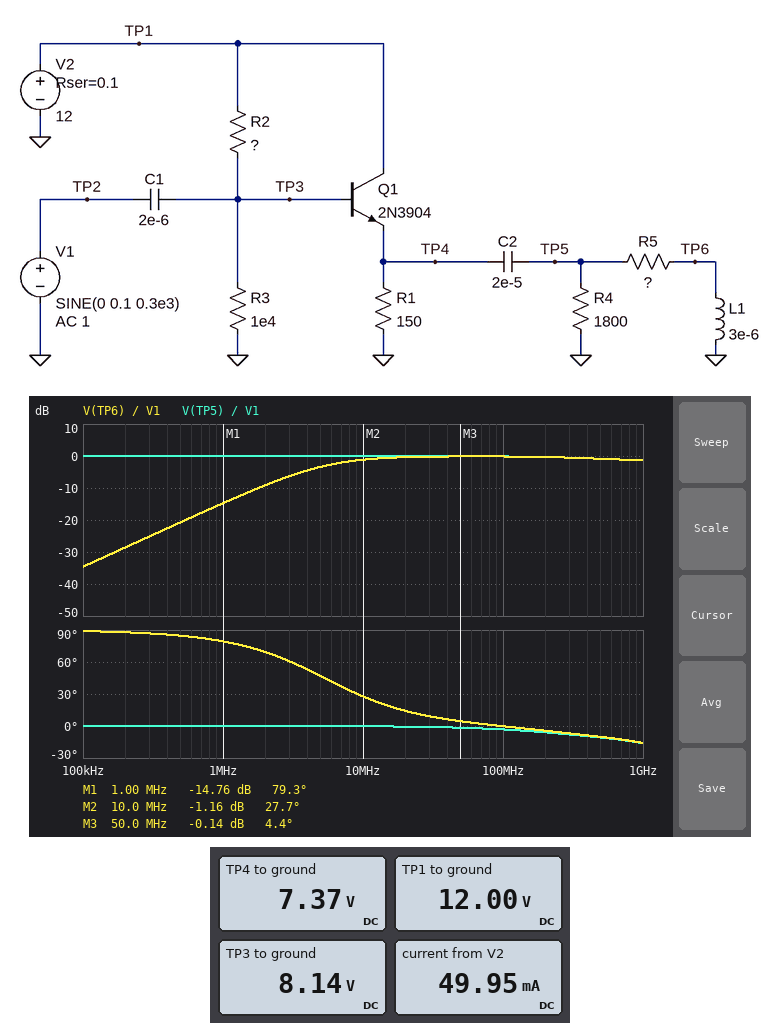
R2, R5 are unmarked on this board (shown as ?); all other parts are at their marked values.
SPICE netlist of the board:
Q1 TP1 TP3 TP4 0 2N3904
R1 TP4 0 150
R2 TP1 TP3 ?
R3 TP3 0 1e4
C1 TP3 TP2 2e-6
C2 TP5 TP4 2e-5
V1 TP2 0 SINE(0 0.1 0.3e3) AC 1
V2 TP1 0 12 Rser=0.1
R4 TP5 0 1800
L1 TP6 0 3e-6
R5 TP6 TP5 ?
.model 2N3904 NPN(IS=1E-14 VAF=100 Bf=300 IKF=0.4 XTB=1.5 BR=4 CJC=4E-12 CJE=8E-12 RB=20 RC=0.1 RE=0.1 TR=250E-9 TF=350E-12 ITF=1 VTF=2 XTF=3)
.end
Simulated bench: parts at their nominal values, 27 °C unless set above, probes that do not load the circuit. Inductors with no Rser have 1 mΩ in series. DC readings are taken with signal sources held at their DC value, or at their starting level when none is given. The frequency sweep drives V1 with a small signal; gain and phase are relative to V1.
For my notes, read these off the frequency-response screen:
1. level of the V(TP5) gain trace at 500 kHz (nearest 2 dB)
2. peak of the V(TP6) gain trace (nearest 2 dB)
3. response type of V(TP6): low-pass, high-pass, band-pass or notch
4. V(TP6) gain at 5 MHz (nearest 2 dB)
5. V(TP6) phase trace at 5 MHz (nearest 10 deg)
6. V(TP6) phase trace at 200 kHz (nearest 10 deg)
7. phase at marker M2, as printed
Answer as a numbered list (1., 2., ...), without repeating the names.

1. 0 dB
2. 0 dB
3. high-pass
4. -4 dB
5. 50 deg
6. 90 deg
7. 27.7 deg
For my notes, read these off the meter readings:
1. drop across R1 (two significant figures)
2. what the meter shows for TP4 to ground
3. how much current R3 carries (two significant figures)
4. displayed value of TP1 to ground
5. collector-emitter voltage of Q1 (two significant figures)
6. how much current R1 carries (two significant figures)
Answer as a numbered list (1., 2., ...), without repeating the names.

1. 7.4 V
2. 7.37 V
3. 810 µA
4. 12.00 V
5. 4.6 V
6. 49 mA
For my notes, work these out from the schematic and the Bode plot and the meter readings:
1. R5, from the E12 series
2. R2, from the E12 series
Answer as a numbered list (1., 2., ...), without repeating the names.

1. 100 Ω
2. 3.9 kΩ
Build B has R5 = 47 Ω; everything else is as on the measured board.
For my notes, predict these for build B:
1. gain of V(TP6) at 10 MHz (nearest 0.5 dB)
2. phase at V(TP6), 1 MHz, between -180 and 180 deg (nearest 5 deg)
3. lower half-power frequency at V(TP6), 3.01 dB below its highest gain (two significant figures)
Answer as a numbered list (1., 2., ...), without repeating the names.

1. -0.5 dB
2. 70 deg
3. 2.5 MHz
